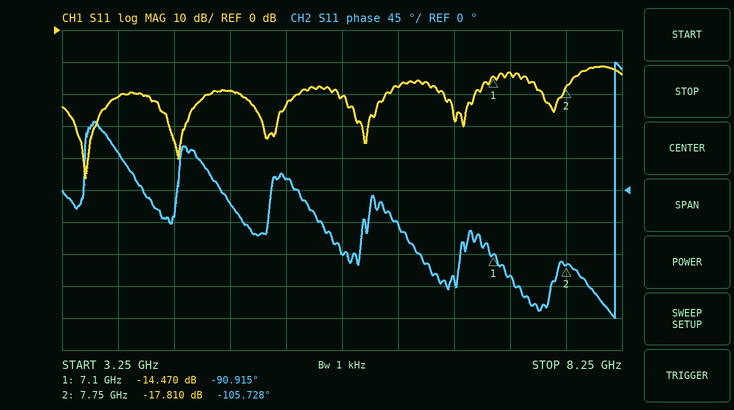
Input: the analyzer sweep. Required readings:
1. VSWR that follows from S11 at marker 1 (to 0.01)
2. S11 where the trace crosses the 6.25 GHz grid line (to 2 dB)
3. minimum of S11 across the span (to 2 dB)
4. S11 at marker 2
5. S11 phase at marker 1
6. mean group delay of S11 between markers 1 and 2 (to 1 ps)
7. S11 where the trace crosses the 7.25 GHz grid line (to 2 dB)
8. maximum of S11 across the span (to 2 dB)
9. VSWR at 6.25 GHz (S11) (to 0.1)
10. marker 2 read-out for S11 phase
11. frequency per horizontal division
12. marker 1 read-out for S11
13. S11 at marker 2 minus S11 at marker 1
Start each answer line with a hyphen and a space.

- 1.47
- -18 dB
- -46 dB
- -17.810 dB
- -90.915°
- 63 ps
- -14 dB
- -12 dB
- 1.3
- -105.728°
- 500 MHz
- -14.470 dB
- -3.340 dB
